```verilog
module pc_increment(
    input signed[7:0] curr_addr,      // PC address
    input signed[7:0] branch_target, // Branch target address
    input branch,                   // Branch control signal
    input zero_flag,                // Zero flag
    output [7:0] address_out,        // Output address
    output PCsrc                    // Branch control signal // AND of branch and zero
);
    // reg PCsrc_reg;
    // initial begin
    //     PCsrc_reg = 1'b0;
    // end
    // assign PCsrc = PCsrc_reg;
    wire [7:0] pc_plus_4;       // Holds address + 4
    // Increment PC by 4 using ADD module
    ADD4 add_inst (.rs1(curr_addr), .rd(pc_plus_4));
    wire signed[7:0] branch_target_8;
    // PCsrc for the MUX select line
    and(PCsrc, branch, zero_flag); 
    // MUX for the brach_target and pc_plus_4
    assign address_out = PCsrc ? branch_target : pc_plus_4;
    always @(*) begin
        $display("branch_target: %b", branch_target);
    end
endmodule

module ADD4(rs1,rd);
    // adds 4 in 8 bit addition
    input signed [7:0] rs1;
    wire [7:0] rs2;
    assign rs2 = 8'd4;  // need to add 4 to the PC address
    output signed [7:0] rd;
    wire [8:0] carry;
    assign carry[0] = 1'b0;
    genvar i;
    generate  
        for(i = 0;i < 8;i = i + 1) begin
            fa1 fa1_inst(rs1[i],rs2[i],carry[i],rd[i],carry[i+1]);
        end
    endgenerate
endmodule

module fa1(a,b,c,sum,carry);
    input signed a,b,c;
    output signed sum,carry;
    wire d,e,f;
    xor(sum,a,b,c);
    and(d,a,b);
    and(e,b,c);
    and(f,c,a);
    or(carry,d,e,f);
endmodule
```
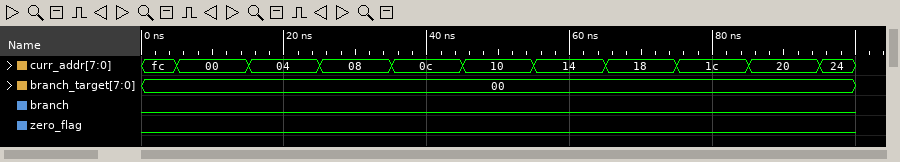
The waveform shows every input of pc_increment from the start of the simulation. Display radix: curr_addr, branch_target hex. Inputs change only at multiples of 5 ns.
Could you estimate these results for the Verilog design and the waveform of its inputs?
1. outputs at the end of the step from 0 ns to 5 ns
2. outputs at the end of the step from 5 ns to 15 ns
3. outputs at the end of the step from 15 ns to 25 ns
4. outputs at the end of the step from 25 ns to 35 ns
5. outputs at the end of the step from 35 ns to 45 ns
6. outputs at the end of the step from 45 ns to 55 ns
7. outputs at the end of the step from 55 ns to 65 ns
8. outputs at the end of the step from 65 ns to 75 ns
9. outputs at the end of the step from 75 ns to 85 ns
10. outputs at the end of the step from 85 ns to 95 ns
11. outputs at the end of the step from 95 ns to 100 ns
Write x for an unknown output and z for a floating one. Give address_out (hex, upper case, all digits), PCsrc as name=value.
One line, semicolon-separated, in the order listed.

address_out=00, PCsrc=0; address_out=04, PCsrc=0; address_out=08, PCsrc=0; address_out=0C, PCsrc=0; address_out=10, PCsrc=0; address_out=14, PCsrc=0; address_out=18, PCsrc=0; address_out=1C, PCsrc=0; address_out=20, PCsrc=0; address_out=24, PCsrc=0; address_out=28, PCsrc=0
